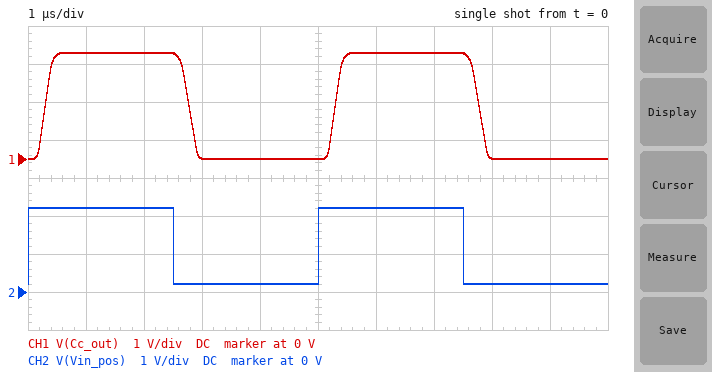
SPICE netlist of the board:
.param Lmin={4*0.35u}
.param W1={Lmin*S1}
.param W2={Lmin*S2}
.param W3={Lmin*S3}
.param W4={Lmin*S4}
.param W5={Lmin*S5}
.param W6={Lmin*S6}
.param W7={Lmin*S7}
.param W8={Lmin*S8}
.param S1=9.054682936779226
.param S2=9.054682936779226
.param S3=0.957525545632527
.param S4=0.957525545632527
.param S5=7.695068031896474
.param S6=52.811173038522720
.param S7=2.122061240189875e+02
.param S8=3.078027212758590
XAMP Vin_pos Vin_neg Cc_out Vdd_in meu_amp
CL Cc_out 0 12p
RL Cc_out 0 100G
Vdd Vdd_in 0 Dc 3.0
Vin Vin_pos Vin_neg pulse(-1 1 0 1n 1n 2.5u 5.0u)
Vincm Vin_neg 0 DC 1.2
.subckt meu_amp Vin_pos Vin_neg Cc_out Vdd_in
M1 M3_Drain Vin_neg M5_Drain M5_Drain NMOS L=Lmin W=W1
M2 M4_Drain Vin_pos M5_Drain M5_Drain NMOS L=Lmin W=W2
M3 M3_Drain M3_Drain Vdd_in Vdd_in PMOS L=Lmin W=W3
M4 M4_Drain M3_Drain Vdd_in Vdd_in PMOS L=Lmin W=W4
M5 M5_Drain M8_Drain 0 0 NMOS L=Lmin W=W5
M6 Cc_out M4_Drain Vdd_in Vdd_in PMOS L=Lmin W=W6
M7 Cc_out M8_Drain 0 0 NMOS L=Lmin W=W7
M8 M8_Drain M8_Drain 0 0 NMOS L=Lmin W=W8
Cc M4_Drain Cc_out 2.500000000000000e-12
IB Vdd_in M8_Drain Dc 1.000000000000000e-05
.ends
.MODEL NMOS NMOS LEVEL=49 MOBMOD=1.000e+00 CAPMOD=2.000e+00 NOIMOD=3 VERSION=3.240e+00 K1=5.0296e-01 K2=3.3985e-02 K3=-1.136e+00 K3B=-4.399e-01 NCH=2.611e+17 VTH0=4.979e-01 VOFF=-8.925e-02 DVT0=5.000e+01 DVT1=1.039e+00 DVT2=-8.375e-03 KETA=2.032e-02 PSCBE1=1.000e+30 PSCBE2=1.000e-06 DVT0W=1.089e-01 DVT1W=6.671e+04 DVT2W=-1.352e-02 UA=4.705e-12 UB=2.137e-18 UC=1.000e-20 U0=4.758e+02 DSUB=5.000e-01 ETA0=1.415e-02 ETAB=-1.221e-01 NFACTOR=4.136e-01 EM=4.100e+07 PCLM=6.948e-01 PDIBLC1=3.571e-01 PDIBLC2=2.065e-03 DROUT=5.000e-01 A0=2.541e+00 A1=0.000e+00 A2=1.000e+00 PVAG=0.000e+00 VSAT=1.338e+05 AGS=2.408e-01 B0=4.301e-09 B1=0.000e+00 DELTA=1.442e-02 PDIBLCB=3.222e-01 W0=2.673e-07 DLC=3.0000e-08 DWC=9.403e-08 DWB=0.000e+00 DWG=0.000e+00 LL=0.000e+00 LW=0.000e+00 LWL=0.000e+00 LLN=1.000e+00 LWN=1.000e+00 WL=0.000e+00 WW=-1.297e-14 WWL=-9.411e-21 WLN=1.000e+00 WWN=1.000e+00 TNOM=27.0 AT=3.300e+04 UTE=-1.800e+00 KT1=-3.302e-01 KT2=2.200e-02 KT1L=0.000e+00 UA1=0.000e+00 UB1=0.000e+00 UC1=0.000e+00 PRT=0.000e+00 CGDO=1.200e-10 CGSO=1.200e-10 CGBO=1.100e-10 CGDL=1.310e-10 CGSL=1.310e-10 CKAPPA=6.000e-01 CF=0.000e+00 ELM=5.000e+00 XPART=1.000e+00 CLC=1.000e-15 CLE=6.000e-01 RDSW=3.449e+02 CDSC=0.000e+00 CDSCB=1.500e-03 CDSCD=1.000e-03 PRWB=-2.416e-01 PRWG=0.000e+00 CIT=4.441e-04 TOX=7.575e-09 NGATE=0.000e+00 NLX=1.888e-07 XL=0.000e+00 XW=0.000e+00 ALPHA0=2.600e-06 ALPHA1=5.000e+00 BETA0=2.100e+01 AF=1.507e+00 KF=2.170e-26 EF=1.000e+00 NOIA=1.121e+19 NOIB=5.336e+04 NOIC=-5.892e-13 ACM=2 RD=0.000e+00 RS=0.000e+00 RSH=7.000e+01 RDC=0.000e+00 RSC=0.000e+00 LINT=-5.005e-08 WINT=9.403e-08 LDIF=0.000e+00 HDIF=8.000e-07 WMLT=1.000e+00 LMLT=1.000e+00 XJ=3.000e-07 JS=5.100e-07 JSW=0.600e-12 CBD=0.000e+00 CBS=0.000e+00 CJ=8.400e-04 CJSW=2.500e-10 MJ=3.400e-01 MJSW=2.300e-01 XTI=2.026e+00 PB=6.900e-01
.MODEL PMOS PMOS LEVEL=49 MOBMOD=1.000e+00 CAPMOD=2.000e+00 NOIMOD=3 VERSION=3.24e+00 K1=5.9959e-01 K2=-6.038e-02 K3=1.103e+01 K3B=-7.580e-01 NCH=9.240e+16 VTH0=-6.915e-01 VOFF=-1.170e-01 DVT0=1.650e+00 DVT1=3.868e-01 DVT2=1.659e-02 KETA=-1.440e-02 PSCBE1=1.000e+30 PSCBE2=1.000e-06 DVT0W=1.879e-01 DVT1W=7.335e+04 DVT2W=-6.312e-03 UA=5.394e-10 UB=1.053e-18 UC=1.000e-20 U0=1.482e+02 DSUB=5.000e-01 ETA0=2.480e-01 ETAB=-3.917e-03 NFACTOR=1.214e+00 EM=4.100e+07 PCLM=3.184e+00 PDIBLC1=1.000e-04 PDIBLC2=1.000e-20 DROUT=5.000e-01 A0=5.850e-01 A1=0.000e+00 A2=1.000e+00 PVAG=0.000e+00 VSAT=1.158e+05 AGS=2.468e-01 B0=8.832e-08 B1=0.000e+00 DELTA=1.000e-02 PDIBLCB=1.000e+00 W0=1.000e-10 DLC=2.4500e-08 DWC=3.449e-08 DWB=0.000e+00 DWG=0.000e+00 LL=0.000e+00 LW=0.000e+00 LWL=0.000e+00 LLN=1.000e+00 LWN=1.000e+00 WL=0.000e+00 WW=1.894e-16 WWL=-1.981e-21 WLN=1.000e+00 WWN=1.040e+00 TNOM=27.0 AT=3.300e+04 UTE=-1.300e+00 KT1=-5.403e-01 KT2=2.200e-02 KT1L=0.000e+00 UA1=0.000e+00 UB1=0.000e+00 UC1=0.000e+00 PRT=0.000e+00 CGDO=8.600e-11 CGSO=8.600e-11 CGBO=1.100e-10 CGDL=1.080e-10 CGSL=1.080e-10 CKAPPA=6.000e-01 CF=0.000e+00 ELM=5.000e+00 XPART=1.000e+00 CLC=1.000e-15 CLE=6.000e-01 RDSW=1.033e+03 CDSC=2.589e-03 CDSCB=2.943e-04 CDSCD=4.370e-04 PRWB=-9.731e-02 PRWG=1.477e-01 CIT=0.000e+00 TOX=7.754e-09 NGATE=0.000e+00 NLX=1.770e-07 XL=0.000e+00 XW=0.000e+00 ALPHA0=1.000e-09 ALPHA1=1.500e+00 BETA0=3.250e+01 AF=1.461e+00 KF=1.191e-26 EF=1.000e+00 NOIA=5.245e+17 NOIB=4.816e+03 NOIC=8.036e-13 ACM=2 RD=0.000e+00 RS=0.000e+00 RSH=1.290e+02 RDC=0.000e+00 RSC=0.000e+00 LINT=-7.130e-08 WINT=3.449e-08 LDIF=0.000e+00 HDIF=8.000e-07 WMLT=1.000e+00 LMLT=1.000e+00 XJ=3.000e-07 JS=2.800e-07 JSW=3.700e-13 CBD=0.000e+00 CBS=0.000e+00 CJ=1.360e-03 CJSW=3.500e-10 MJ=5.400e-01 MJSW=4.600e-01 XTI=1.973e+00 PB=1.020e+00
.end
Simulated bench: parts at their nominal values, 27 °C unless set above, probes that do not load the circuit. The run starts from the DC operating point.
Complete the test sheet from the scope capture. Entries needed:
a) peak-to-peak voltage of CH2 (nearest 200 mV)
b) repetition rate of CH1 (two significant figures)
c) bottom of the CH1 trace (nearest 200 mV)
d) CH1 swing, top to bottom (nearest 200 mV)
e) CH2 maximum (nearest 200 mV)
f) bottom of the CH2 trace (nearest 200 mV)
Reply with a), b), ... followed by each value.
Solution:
a) 2.0 V
b) 200 kHz
c) 0 V
d) 2.8 V
e) 2.2 V
f) 200 mV
